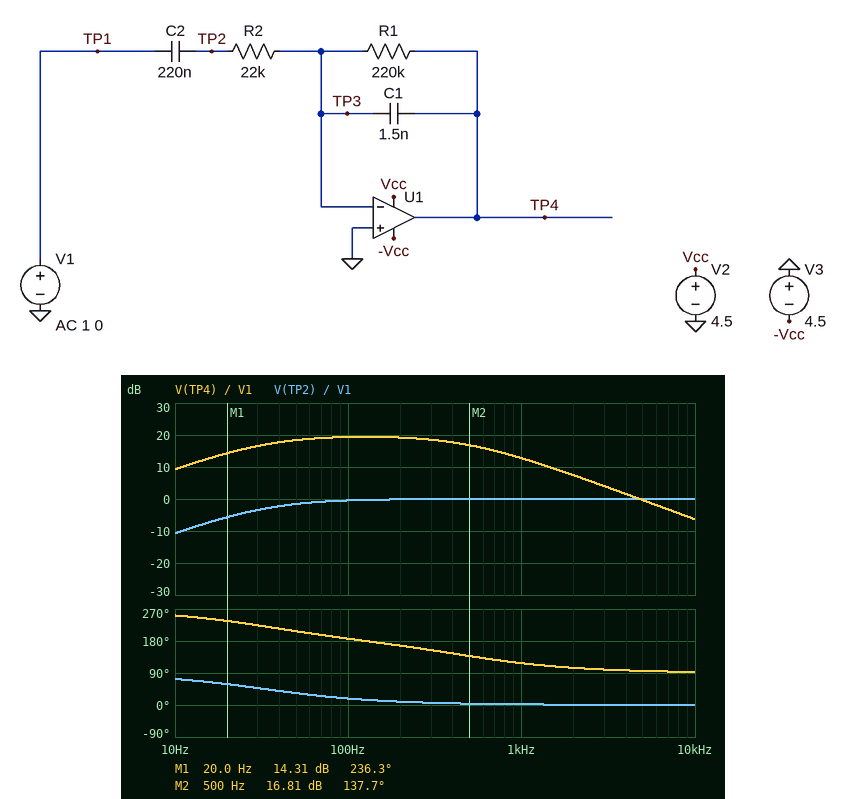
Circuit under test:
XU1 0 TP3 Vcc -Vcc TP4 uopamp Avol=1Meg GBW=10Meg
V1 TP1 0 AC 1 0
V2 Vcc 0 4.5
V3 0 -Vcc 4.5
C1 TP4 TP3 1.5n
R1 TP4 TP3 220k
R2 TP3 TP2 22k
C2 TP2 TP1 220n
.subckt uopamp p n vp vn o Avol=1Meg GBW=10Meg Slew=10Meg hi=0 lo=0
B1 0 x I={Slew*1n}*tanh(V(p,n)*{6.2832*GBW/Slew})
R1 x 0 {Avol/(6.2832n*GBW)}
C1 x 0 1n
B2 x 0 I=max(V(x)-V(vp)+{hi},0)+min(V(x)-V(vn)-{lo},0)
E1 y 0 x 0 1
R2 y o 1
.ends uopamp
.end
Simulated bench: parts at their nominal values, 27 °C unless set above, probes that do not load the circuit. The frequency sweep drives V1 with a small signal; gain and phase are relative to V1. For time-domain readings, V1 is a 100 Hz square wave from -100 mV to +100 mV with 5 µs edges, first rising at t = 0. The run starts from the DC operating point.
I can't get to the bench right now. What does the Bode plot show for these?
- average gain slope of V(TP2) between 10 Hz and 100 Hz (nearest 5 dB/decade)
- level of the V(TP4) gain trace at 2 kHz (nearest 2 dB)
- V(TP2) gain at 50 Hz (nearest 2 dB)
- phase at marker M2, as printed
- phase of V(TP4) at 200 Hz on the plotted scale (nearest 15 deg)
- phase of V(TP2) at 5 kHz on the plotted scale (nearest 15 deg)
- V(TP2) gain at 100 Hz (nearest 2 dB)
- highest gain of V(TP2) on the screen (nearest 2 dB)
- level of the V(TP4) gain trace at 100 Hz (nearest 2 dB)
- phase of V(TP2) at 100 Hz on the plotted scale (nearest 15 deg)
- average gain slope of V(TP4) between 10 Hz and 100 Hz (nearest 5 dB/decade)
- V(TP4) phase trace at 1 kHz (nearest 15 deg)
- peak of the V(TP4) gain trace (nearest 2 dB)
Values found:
10 dB/decade
8 dB
-2 dB
137.7 deg
165 deg
0 deg
0 dB
0 dB
20 dB
15 deg
10 dB/decade
120 deg
20 dB
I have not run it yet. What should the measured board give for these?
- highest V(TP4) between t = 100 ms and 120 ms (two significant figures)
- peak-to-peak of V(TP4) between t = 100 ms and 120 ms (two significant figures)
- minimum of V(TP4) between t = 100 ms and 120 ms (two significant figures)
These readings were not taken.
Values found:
1.2 V
2.4 V
-1.2 V
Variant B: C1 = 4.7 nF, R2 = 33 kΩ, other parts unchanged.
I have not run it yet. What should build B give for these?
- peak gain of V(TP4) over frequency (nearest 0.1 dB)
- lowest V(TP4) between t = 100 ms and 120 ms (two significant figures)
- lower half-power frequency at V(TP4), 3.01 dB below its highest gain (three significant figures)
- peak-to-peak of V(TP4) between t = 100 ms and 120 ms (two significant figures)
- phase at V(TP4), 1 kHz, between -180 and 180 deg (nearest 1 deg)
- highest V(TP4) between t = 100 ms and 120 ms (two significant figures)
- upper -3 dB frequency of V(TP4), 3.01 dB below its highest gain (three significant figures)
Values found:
15.3 dB
-600 mV
17.5 Hz
1.2 V
100 deg
600 mV
193 Hz
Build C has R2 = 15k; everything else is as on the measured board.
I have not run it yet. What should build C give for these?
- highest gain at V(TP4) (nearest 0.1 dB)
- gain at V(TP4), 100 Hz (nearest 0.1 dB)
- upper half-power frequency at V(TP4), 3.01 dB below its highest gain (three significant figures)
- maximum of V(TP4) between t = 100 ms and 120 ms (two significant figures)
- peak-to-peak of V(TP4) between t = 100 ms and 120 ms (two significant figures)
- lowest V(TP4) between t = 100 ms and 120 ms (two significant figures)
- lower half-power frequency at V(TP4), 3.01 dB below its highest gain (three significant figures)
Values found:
22.5 dB
22.2 dB
571 Hz
1.8 V
3.6 V
-1.8 V
40.7 Hz
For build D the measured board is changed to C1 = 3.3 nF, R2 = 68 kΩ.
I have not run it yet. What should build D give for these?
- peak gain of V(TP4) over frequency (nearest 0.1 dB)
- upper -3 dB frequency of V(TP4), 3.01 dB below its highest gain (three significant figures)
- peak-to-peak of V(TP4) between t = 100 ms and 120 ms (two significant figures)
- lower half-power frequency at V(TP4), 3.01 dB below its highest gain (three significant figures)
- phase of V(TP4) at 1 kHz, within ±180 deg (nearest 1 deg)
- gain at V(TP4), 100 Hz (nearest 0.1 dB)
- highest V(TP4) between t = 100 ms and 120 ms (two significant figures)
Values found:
9.8 dB
240 Hz
630 mV
9.73 Hz
103 deg
9.3 dB
310 mV
